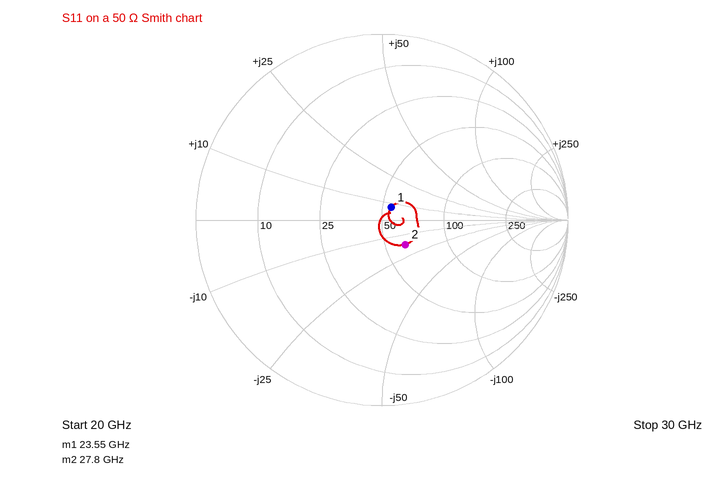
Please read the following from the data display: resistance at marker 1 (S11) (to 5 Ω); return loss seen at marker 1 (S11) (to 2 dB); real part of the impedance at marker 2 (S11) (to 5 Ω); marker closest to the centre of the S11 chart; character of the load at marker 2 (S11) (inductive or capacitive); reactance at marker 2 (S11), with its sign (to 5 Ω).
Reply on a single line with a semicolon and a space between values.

55 Ω; 22 dB; 60 Ω; marker 1; capacitive; -15 Ω
